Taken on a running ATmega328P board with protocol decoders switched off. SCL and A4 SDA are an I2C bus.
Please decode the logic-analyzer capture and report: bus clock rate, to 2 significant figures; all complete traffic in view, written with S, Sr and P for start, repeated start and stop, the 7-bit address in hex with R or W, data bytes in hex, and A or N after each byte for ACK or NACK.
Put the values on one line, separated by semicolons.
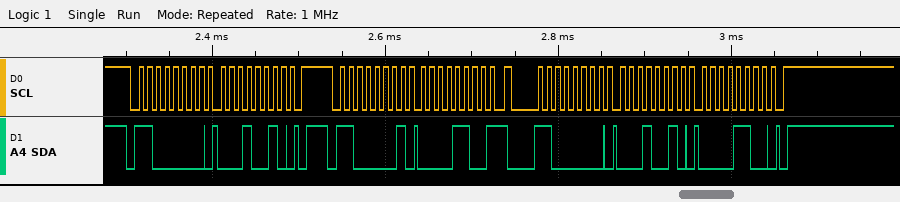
100 kHz; S 60W A 12 A P S 60R A 0C N Sr 60W A 12 A 0C A P
